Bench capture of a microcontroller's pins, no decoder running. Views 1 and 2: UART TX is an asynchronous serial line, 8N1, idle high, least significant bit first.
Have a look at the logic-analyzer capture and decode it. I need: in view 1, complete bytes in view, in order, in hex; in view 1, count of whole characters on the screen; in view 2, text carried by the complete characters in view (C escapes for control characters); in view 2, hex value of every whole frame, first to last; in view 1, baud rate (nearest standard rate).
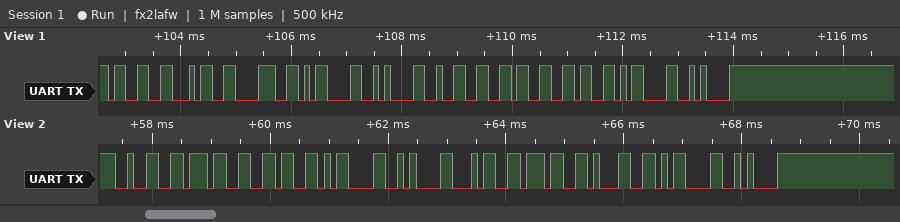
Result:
33 34 38 0D 0A 32 36 36 0D 0A
10
"276\r\n471\r\n"
32 37 36 0D 0A 34 37 31 0D 0A
9600 baud
